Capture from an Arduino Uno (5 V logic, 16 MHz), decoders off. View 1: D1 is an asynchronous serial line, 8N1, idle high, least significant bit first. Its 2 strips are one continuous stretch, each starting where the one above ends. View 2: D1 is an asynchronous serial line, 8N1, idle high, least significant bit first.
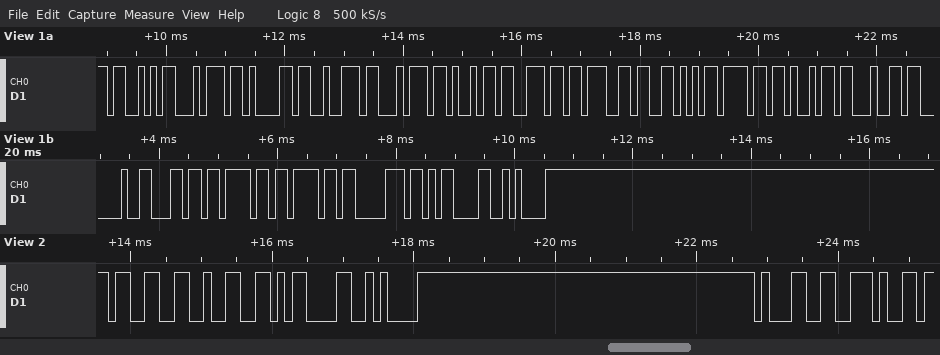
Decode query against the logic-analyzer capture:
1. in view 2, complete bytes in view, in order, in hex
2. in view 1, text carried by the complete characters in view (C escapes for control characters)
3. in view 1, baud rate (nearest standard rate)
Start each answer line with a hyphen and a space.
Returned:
- 0x33 0x32 0x0D 0x0A 0x31 0x2E
- "StartingVoid loop\r\n"
- 9600 baud
